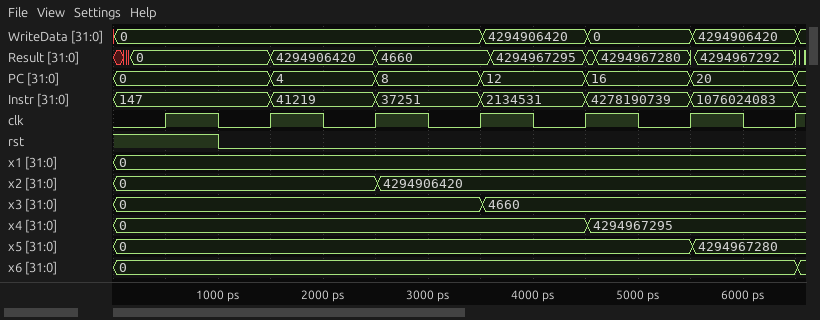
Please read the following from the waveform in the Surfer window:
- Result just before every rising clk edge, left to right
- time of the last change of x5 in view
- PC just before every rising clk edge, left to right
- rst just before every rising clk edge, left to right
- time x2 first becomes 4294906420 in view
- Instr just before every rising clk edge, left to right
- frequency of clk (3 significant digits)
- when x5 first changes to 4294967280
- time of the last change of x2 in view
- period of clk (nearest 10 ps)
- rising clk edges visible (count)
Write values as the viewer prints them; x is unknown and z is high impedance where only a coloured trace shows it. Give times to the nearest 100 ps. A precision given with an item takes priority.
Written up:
0, 0, 4294906420, 4660, 4294967295, 4294967280, 4294967292
5500 ps
0, 0, 4, 8, 12, 16, 20
1 0 0 0 0 0 0
2500 ps
147, 147, 41219, 37251, 2134531, 4278190739, 1076024083
1.00 GHz
5500 ps
2500 ps
1000 ps
7
